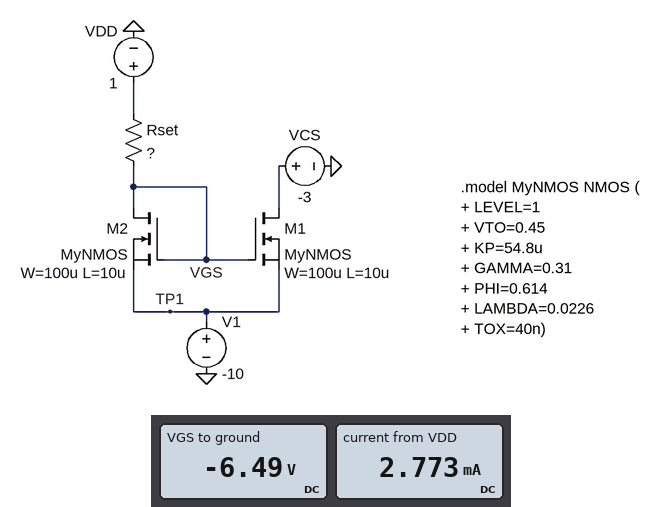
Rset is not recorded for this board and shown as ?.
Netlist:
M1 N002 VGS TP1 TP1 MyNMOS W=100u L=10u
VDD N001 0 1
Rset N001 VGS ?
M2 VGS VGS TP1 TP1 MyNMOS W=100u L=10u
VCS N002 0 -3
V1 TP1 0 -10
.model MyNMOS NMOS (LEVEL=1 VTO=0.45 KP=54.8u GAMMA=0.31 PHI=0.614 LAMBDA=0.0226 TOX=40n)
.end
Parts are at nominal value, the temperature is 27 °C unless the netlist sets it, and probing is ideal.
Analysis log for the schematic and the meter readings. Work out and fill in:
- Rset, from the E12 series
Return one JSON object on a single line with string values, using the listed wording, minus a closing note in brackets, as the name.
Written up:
{"Rset, from the E12 series": "2.7 kΩ"}
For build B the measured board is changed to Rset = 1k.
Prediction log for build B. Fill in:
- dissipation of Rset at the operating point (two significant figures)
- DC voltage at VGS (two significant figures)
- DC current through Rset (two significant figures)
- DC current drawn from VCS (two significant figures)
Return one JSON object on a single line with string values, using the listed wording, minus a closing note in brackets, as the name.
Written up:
{"dissipation of Rset at the operating point": "37 mW", "DC voltage at VGS": "-5.1 V", "DC current through Rset": "6.1 mA", "DC current drawn from VCS": "6.3 mA"}
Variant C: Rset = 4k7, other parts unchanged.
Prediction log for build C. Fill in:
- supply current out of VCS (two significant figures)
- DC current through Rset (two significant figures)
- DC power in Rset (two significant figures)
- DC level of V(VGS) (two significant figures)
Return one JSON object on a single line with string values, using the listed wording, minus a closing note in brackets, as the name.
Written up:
{"supply current out of VCS": "1.9 mA", "DC current through Rset": "1.7 mA", "DC power in Rset": "14 mW", "DC level of V(VGS)": "-7.1 V"}
